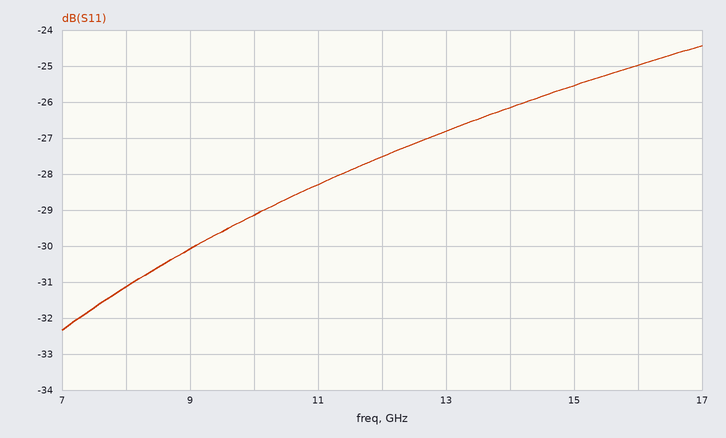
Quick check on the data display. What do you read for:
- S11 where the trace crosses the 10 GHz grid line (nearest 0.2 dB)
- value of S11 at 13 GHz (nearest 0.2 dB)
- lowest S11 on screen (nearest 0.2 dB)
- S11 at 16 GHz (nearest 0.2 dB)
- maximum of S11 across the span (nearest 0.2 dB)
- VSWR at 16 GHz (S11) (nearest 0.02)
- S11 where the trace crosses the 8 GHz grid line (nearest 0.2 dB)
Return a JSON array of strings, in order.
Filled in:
["-29.2 dB", "-26.8 dB", "-32.4 dB", "-25.0 dB", "-24.4 dB", "1.12", "-31.2 dB"]
